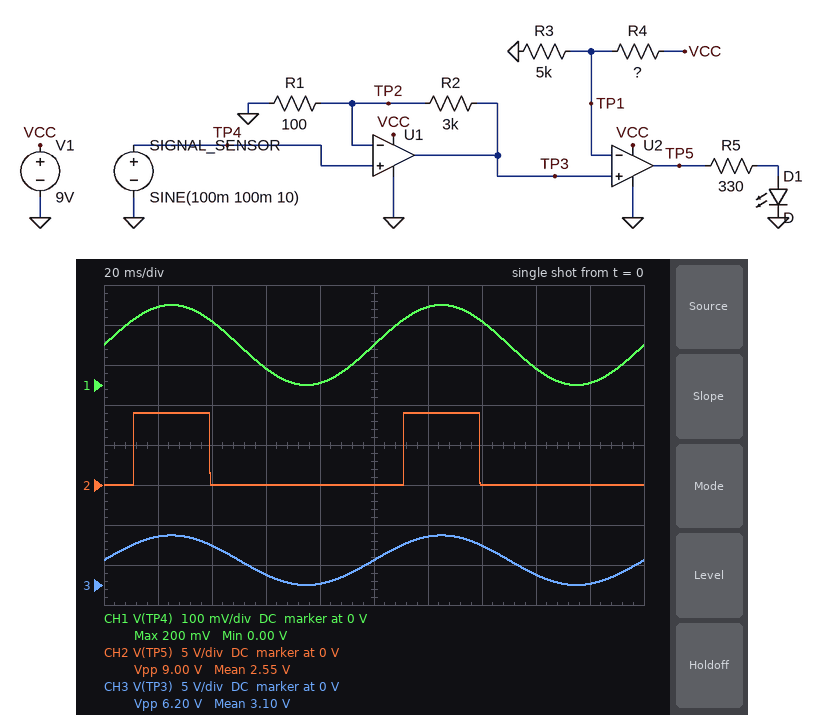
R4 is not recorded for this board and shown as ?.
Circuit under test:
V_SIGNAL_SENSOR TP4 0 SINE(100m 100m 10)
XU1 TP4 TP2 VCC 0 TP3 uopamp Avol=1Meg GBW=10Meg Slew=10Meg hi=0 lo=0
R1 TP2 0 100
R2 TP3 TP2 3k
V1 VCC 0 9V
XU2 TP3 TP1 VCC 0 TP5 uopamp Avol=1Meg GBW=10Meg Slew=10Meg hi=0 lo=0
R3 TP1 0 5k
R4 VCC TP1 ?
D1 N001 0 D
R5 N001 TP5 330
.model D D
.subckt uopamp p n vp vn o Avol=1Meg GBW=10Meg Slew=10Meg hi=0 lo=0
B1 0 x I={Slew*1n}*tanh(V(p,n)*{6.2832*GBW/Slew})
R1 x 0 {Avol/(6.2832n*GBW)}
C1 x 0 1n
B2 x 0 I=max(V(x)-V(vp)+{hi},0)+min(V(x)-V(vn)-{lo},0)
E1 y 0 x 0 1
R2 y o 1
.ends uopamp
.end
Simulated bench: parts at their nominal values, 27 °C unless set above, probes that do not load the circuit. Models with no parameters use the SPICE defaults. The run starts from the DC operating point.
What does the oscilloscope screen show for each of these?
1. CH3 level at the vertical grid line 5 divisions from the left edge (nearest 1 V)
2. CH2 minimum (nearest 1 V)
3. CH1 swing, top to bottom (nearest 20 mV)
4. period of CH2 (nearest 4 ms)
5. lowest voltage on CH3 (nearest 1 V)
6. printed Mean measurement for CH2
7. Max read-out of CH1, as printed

3 V
0 V
200 mV
100 ms
0 V
2.55 V
200 mV
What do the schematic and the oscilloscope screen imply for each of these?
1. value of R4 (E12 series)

3.9 kΩ
